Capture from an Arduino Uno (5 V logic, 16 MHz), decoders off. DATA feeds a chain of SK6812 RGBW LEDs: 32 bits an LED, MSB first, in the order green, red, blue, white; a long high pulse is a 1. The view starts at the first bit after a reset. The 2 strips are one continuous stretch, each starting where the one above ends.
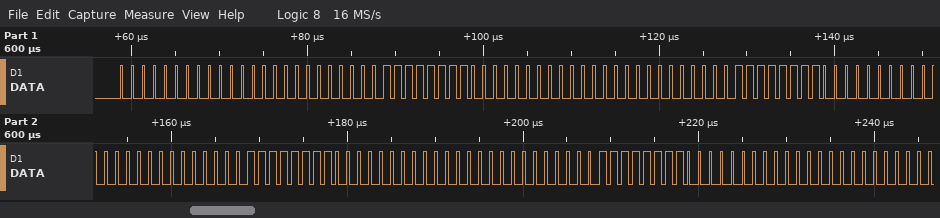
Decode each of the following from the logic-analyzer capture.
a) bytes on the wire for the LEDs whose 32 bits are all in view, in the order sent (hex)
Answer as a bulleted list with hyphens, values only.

- 00 00 00 FF 00 00 00 FF 00 00 00 FF 00 00 00 FF
